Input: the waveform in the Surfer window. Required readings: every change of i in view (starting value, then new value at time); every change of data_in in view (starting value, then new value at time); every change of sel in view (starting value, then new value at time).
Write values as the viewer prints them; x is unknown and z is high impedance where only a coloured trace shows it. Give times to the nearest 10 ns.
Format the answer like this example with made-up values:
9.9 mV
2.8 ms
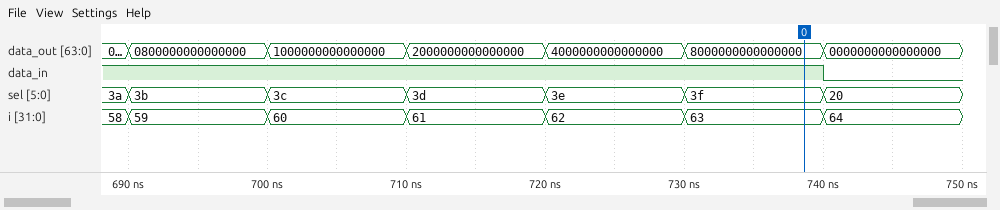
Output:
58, 59 at 690 ns, 60 at 700 ns, 61 at 710 ns, 62 at 720 ns, 63 at 730 ns, 64 at 740 ns
1, 0 at 740 ns
3a, 3b at 690 ns, 3c at 700 ns, 3d at 710 ns, 3e at 720 ns, 3f at 730 ns, 20 at 740 ns
